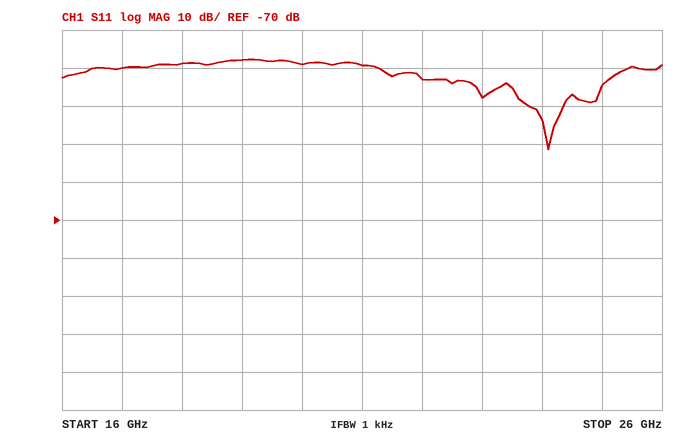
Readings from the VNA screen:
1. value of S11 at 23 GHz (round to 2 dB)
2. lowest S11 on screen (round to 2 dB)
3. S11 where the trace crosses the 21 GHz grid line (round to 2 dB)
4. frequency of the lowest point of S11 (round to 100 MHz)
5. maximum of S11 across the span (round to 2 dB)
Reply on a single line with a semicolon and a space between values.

-38 dB; -52 dB; -30 dB; 24.1 GHz; -28 dB
